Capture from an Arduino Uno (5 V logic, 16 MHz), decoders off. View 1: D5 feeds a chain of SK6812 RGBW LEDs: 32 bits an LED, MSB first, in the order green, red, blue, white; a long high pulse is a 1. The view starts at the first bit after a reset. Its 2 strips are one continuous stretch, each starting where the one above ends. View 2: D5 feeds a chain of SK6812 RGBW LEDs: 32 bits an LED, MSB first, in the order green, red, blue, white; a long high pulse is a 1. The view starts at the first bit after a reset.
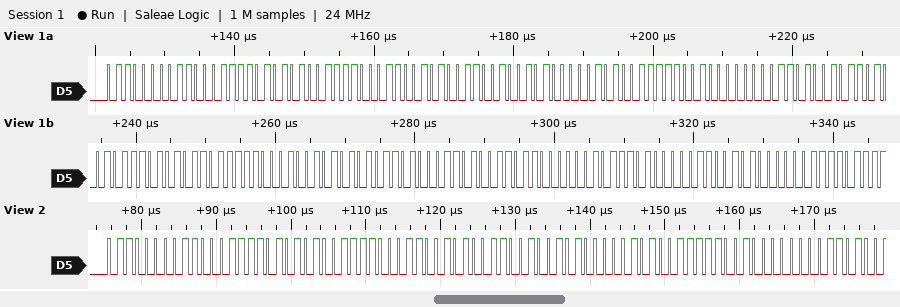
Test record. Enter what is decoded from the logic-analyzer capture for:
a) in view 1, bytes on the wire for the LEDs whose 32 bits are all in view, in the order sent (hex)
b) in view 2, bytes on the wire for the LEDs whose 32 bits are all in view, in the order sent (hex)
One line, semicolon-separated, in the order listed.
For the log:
60 C7 AA 78 CA 64 A0 A7 C8 06 96 97 56 F8 95 5A 34 D8 17 41; 60 C7 AA 78 CA 64 A0 A7
